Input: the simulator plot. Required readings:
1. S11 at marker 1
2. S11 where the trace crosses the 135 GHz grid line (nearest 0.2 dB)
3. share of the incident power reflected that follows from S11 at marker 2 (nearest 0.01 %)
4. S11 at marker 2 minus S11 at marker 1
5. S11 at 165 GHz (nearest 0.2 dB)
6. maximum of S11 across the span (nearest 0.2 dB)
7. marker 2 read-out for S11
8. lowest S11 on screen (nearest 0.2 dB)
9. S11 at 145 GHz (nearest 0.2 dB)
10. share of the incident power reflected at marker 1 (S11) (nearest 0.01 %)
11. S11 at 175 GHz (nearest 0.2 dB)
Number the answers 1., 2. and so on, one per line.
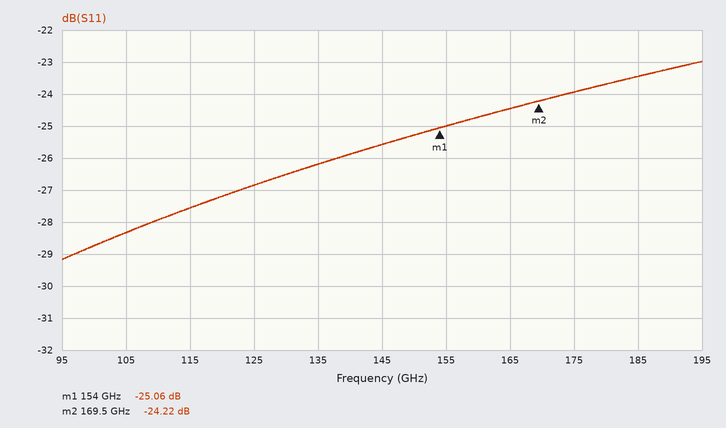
1. -25.06 dB
2. -26.2 dB
3. 0.38 %
4. 0.84 dB
5. -24.4 dB
6. -23.0 dB
7. -24.22 dB
8. -29.2 dB
9. -25.6 dB
10. 0.31 %
11. -24.0 dB
